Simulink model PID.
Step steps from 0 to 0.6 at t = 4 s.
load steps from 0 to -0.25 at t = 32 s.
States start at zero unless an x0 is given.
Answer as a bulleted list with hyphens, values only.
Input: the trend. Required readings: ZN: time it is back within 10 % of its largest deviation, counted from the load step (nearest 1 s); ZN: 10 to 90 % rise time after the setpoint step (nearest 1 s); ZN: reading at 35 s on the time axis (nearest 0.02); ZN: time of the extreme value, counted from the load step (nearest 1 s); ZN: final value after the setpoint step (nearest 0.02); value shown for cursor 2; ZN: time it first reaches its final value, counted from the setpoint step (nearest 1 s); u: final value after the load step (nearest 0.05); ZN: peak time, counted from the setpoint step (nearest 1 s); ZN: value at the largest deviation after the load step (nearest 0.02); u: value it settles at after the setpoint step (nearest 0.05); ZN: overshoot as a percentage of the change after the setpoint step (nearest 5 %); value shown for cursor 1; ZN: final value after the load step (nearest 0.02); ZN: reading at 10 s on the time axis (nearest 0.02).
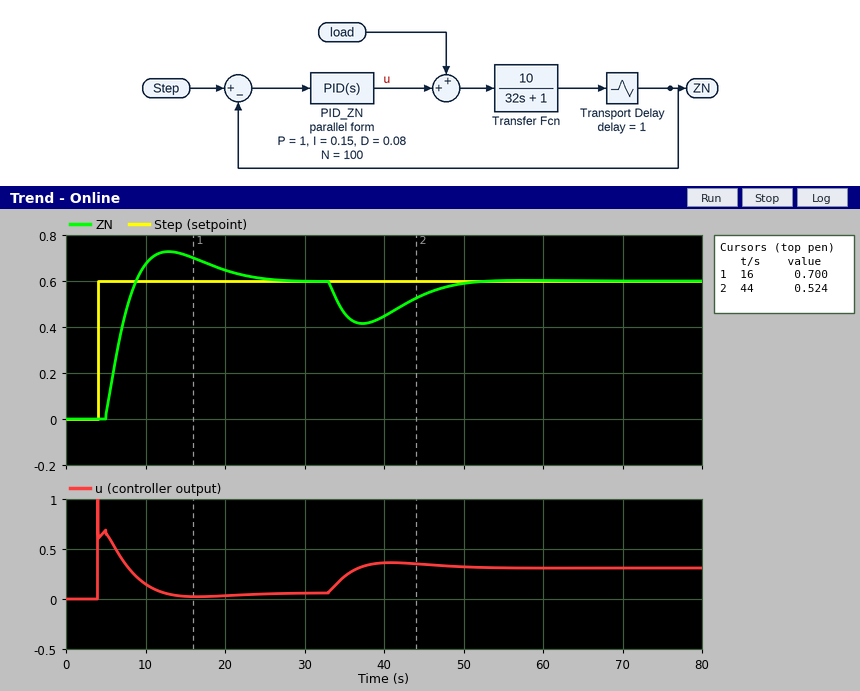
- 17 s
- 3 s
- 0.46
- 5 s
- 0.60
- 0.524
- 5 s
- 0.30
- 9 s
- 0.42
- 0.05
- 20 %
- 0.700
- 0.60
- 0.68
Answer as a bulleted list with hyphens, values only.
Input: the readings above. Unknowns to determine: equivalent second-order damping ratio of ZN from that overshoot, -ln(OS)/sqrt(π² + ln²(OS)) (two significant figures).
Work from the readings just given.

- 0.46
